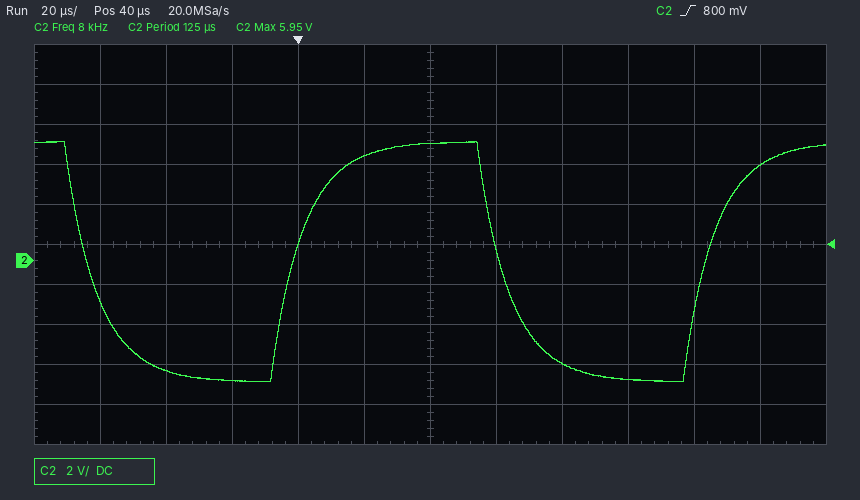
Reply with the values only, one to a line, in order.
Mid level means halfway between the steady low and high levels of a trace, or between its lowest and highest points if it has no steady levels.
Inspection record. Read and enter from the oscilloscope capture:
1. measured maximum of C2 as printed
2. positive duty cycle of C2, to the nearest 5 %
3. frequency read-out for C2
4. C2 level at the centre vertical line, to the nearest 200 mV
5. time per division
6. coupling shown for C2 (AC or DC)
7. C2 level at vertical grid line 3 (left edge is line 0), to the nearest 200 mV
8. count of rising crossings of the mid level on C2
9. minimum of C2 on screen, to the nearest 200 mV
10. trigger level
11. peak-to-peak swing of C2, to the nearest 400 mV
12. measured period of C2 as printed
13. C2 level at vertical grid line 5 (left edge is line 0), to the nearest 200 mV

5.95 V
50 %
8 kHz
5.8 V
20 µs
DC
-6.0 V
2
-6.0 V
800 mV
12.0 V
125 µs
5.2 V
